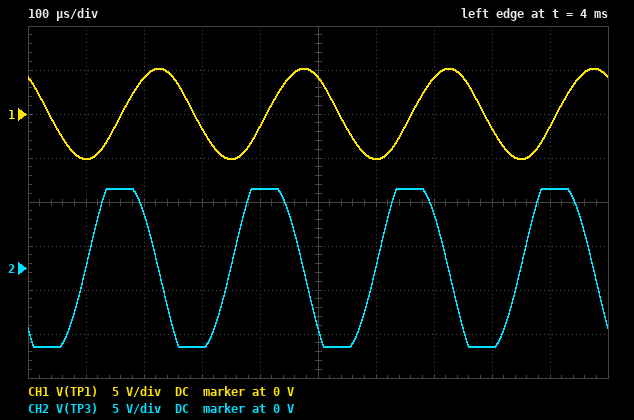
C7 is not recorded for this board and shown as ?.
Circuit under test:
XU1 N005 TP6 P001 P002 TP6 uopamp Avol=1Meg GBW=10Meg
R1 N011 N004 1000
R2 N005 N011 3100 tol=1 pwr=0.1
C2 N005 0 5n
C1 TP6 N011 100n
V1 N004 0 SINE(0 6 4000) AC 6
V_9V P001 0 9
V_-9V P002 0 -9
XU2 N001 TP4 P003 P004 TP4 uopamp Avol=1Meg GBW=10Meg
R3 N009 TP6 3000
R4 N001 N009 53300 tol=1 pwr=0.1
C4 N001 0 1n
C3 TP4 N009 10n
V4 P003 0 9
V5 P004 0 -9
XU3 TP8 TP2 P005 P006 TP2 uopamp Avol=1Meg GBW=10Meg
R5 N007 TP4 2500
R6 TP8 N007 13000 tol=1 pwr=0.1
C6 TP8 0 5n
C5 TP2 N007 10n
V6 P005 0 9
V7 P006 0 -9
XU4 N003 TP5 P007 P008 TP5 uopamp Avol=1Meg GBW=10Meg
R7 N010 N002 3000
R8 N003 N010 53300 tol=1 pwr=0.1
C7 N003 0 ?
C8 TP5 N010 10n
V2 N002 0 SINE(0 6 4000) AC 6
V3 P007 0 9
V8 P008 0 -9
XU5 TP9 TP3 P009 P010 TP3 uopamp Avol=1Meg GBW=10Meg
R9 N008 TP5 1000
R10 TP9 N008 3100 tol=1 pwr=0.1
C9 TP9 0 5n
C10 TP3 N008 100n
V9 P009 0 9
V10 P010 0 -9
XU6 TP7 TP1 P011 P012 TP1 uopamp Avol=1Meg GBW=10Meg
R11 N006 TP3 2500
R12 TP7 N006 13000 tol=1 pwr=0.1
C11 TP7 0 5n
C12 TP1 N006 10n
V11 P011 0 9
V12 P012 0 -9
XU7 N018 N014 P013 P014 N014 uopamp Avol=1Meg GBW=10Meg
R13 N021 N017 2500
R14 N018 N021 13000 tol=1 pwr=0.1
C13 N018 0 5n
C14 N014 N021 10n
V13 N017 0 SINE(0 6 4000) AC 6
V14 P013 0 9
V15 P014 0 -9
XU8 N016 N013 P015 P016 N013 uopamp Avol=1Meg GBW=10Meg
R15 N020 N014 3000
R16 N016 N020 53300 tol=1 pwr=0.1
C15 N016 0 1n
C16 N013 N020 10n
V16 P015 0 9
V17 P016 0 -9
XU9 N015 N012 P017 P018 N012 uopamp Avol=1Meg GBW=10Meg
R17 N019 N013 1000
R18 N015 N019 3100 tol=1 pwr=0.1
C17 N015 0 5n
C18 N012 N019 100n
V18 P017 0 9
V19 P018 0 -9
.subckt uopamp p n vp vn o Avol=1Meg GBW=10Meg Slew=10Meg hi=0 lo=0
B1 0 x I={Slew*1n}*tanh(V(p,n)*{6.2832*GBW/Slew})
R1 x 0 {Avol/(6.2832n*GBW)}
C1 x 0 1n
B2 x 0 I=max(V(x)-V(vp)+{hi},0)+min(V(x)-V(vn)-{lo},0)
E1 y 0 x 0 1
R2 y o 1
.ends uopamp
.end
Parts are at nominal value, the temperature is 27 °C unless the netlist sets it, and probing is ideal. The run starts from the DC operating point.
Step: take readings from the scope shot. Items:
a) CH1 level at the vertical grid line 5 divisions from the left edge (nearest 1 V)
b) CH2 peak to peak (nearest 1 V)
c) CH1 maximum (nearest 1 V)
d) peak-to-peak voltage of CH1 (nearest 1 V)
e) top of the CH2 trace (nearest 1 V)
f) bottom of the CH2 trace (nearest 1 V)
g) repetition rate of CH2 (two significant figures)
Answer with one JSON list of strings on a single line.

["4 V", "18 V", "5 V", "10 V", "9 V", "-9 V", "4.0 kHz"]
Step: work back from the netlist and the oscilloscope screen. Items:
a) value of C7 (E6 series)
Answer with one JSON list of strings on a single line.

["470 pF"]
